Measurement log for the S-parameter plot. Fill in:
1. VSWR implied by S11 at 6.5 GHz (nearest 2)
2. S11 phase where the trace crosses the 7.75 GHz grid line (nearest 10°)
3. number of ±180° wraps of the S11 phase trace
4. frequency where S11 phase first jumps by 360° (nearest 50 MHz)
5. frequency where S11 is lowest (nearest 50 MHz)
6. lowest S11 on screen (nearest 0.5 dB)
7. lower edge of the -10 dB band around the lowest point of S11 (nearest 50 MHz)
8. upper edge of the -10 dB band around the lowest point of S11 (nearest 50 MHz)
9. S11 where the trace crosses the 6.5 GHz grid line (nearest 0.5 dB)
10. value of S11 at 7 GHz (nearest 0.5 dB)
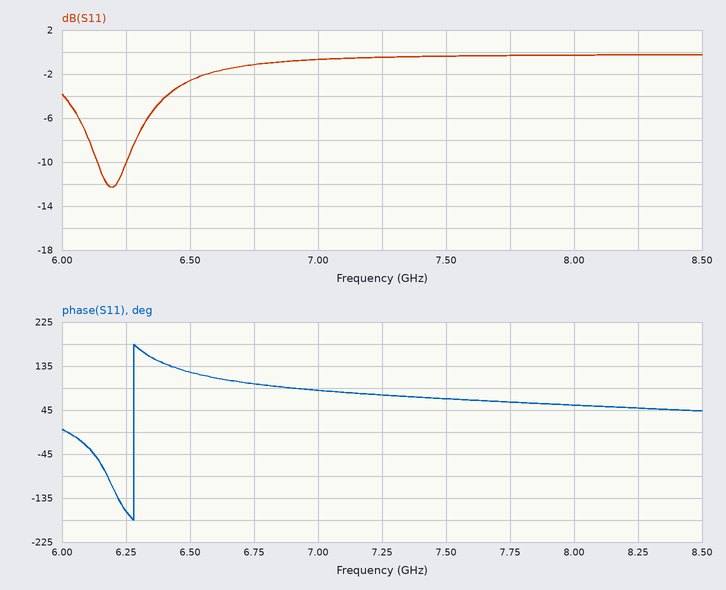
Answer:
6
60°
1
6.30 GHz
6.20 GHz
-12.5 dB
6.15 GHz
6.25 GHz
-2.5 dB
-0.5 dB
